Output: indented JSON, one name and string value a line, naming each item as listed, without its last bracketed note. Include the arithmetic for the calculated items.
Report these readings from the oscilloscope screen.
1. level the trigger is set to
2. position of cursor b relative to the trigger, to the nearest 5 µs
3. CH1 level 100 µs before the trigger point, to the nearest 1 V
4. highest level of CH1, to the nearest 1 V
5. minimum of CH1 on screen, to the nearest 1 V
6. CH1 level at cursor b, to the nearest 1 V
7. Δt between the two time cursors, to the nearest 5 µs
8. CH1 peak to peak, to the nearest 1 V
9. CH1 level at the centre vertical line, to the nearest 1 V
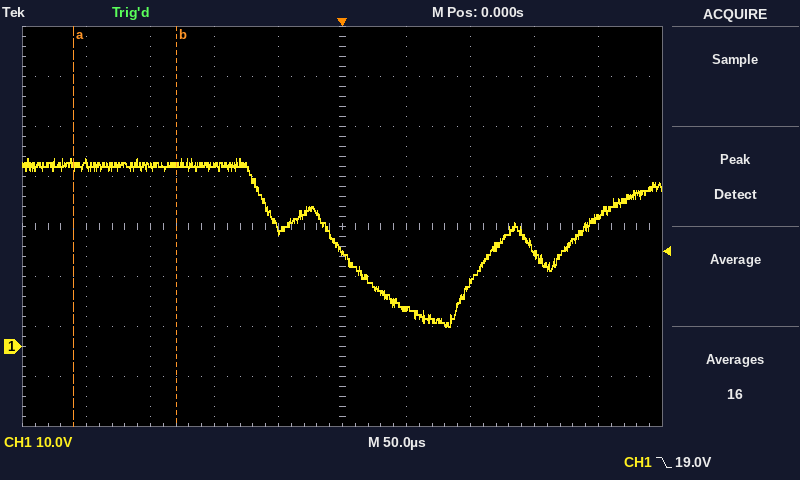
{
  "level the trigger is set to": "19.0 V",
  "position of cursor b relative to the trigger, to the nearest 5 µs": "-130 µs",
  "CH1 level 100 µs before the trigger point, to the nearest 1 V": "36 V",
  "highest level of CH1, to the nearest 1 V": "38 V",
  "minimum of CH1 on screen, to the nearest 1 V": "4 V",
  "CH1 level at cursor b, to the nearest 1 V": "36 V",
  "Δt between the two time cursors, to the nearest 5 µs": "80 µs",
  "CH1 peak to peak, to the nearest 1 V": "38 V − (4 V) = 34 V",
  "CH1 level at the centre vertical line, to the nearest 1 V": "19 V"
}
